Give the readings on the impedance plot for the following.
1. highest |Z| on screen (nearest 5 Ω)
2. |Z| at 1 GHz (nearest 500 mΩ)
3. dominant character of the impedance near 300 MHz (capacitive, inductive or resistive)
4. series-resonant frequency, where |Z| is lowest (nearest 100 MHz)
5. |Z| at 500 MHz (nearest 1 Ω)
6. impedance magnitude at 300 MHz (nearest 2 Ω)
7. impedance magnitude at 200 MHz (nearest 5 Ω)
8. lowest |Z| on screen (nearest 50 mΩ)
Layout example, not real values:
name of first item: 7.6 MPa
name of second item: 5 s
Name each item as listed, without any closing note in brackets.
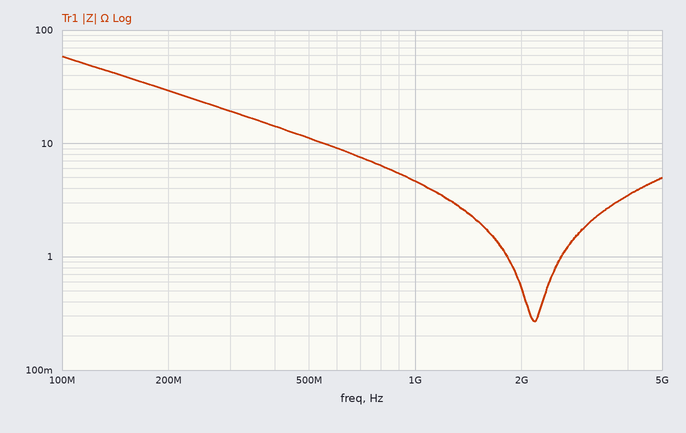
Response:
highest |Z| on screen: 60 Ω
|Z| at 1 GHz: 4.5 Ω
dominant character of the impedance near 300 MHz: capacitive
series-resonant frequency, where |Z| is lowest: 2.2 GHz
|Z| at 500 MHz: 11 Ω
impedance magnitude at 300 MHz: 20 Ω
impedance magnitude at 200 MHz: 30 Ω
lowest |Z| on screen: 250 mΩ
